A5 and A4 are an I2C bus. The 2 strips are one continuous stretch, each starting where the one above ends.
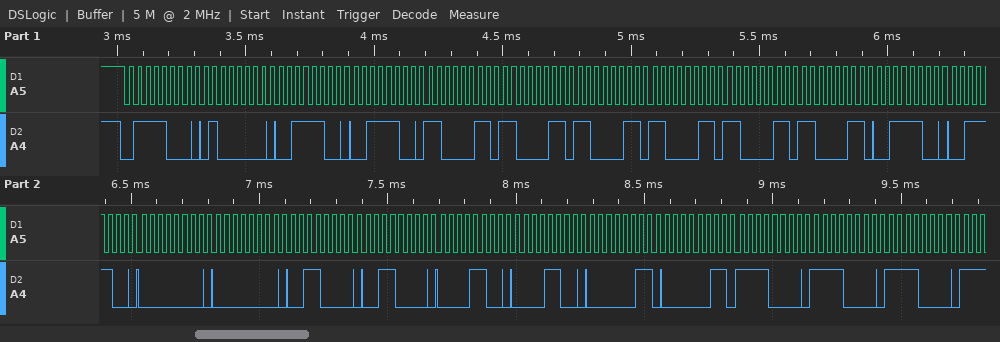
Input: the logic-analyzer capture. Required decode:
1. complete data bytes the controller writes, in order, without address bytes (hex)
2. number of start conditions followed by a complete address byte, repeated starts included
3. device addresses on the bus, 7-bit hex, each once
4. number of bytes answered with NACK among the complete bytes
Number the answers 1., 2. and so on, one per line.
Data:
1. 40 3C 3C C3 C3 C3 C3 C3 C3 3C 3C 00 00 30 30 0C 0C 03 03 F0 F0 F0
2. 1
3. 0x3C
4. 0
